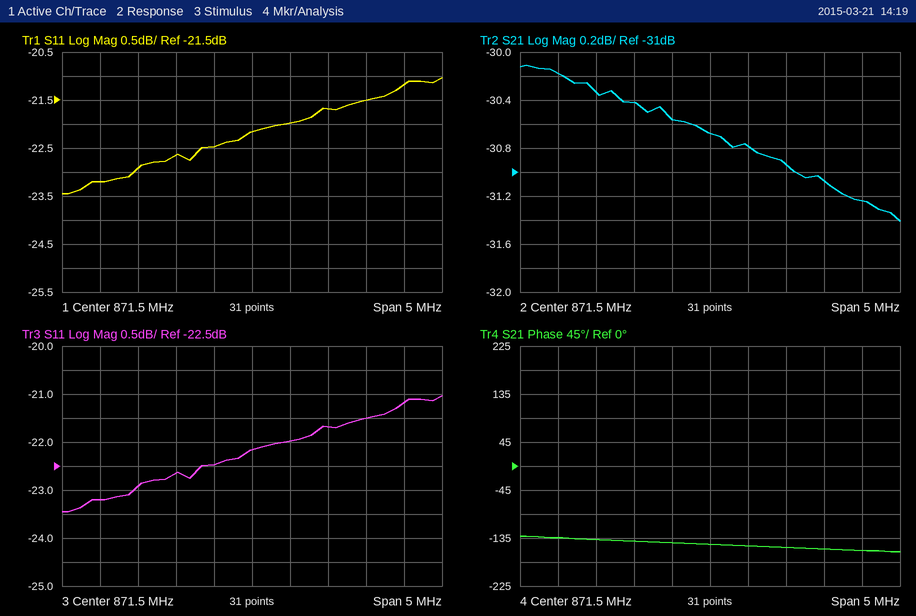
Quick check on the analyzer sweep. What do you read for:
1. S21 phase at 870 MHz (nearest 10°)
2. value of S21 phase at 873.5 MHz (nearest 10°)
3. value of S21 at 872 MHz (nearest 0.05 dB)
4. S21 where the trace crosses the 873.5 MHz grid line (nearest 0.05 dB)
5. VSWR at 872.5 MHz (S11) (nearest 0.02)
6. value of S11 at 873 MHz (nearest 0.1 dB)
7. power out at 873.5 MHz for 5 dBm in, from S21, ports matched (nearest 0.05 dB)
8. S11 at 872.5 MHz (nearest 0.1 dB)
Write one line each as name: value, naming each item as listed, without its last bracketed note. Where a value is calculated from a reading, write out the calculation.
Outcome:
S21 phase at 870 MHz: -140°
value of S21 phase at 873.5 MHz: -160°
value of S21 at 872 MHz: -30.80 dB
S21 where the trace crosses the 873.5 MHz grid line: -31.25 dB
VSWR at 872.5 MHz (S11): |Γ| = 10^(-21.7/20) = 0.0822; VSWR = (1 + 0.0822)/(1 − 0.0822) ≈ 1.18
value of S11 at 873 MHz: -21.5 dB
power out at 873.5 MHz for 5 dBm in, from S21, ports matched: 5 dBm + (-31.25 dB) = -26.25 dBm
S11 at 872.5 MHz: -21.7 dB
